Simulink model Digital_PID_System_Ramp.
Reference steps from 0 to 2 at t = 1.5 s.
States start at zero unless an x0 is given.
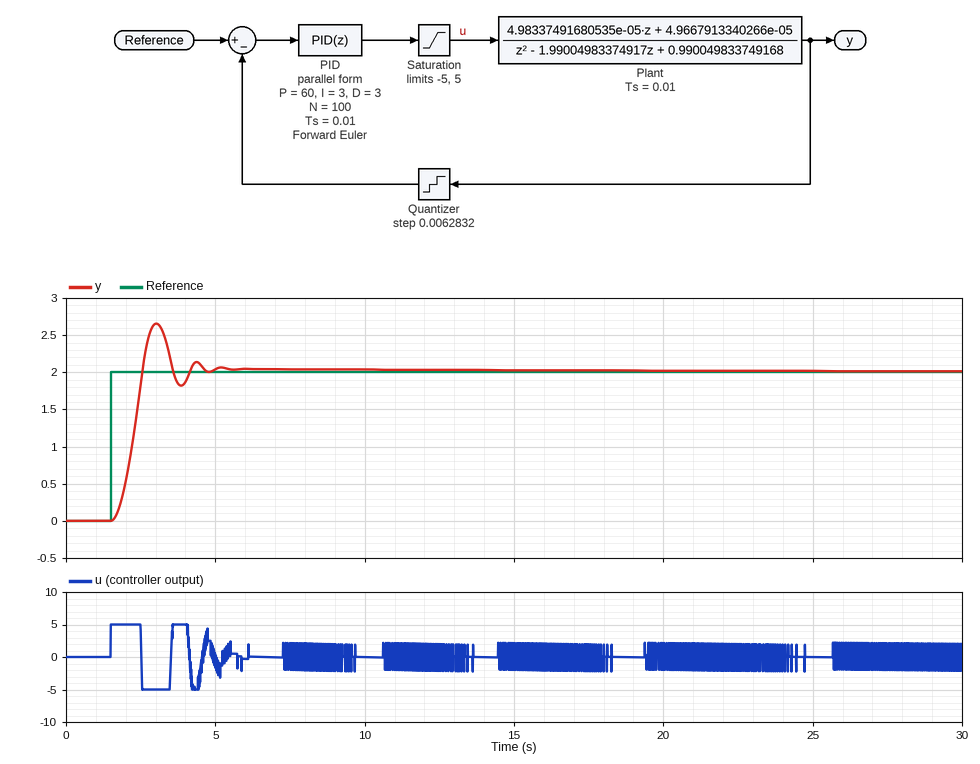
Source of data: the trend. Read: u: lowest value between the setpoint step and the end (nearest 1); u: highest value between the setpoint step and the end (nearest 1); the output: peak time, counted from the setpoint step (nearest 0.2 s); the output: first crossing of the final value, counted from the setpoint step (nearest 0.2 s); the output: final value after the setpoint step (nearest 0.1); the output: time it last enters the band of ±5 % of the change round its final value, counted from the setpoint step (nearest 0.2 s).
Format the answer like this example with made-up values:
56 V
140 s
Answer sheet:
-5
5
1.6 s
1.0 s
2.0
3.0 s
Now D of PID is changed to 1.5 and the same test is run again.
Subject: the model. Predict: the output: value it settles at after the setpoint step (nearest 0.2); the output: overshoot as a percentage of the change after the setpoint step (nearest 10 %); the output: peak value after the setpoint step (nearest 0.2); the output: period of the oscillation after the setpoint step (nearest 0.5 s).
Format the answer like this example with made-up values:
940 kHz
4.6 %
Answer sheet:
2.0
40 %
2.8
1.5 s
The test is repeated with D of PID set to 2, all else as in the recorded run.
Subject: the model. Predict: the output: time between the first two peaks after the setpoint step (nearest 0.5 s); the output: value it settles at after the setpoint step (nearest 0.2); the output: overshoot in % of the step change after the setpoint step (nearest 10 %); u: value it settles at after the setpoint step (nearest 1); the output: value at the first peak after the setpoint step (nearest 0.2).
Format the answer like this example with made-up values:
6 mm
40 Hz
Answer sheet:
1.5 s
2.0
40 %
0
2.8
